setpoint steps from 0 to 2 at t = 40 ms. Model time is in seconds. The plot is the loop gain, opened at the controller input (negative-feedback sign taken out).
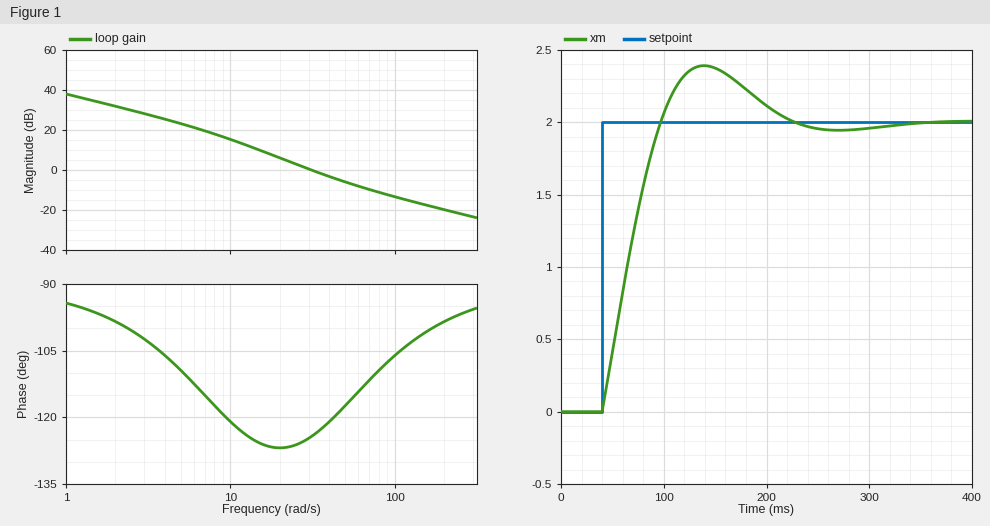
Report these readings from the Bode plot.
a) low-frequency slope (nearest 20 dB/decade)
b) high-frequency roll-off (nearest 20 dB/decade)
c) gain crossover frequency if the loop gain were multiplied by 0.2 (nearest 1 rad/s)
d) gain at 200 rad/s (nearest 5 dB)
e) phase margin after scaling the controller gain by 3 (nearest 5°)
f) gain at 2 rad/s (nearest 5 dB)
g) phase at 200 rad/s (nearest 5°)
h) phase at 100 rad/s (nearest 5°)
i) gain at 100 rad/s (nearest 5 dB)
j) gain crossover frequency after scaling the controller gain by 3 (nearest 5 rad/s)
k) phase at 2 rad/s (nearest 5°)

-20 dB/decade
-20 dB/decade
11 rad/s
-20 dB
70°
30 dB
-100°
-105°
-15 dB
70 rad/s
-100°
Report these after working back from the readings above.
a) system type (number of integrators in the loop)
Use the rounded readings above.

1
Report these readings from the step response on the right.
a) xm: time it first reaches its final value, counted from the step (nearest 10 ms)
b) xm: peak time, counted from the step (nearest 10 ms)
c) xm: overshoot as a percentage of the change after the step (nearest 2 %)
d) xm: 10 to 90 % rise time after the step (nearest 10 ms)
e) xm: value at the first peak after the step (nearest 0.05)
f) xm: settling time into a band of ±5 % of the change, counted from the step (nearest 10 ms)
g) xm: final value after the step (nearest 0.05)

60 ms
100 ms
20 %
40 ms
2.40
160 ms
2.00
